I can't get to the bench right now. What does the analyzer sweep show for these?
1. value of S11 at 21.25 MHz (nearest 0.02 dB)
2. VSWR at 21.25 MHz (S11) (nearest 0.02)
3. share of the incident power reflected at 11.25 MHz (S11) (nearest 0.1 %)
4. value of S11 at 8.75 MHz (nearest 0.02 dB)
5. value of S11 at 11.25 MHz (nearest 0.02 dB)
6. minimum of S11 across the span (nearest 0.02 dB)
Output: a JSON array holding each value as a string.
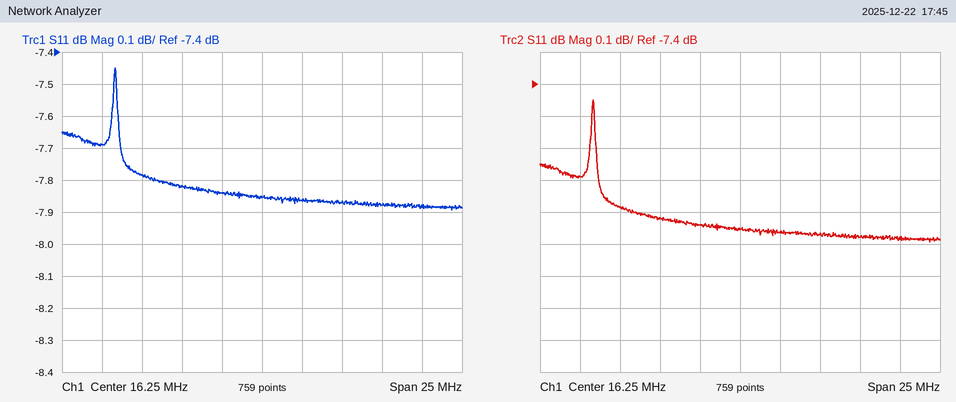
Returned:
["-7.86 dB", "2.36", "16.5 %", "-7.78 dB", "-7.82 dB", "-7.90 dB"]
